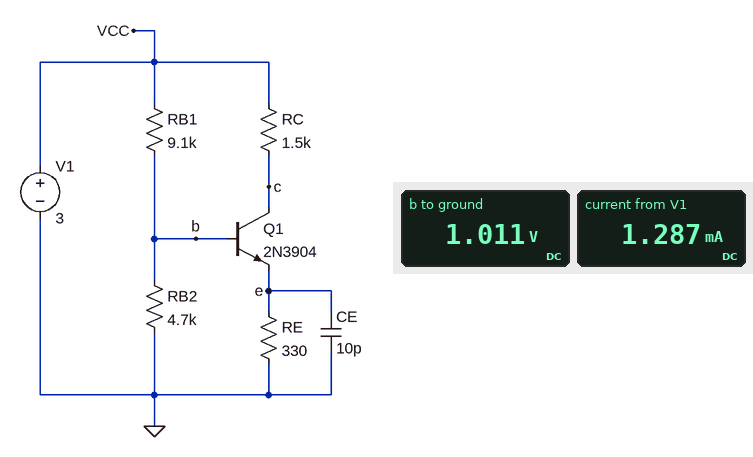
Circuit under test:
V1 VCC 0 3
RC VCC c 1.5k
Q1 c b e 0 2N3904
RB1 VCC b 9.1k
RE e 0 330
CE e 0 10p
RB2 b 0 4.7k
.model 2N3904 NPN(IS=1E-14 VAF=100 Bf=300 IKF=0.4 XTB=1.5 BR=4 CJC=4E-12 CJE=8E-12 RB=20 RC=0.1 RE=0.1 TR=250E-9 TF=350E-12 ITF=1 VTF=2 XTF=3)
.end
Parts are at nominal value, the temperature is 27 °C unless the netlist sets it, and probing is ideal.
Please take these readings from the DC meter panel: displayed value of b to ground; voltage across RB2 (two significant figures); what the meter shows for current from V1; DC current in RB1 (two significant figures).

1.011 V
1.0 V
1.287 mA
220 µA
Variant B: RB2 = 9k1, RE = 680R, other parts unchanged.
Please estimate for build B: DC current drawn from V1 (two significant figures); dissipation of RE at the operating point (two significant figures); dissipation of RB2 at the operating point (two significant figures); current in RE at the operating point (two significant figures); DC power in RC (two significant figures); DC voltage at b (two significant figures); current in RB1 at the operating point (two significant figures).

1.4 mA
990 µW
240 µW
1.2 mA
2.2 mW
1.5 V
170 µA
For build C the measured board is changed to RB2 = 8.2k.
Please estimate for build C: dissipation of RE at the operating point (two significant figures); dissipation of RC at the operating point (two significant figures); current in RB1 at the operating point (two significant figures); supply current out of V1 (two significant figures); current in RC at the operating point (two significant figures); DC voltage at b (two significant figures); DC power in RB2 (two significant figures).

890 µW
3.8 mW
200 µA
1.8 mA
1.6 mA
1.2 V
180 µW
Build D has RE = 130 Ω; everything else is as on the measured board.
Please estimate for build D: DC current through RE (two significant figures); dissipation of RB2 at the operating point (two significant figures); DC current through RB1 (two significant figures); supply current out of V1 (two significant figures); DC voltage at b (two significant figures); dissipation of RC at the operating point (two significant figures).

1.8 mA
180 µW
230 µA
2.0 mA
910 mV
4.8 mW
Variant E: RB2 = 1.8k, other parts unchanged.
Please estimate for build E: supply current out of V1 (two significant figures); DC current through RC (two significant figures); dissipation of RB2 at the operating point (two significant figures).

280 µA
2.1 µA
140 µW
